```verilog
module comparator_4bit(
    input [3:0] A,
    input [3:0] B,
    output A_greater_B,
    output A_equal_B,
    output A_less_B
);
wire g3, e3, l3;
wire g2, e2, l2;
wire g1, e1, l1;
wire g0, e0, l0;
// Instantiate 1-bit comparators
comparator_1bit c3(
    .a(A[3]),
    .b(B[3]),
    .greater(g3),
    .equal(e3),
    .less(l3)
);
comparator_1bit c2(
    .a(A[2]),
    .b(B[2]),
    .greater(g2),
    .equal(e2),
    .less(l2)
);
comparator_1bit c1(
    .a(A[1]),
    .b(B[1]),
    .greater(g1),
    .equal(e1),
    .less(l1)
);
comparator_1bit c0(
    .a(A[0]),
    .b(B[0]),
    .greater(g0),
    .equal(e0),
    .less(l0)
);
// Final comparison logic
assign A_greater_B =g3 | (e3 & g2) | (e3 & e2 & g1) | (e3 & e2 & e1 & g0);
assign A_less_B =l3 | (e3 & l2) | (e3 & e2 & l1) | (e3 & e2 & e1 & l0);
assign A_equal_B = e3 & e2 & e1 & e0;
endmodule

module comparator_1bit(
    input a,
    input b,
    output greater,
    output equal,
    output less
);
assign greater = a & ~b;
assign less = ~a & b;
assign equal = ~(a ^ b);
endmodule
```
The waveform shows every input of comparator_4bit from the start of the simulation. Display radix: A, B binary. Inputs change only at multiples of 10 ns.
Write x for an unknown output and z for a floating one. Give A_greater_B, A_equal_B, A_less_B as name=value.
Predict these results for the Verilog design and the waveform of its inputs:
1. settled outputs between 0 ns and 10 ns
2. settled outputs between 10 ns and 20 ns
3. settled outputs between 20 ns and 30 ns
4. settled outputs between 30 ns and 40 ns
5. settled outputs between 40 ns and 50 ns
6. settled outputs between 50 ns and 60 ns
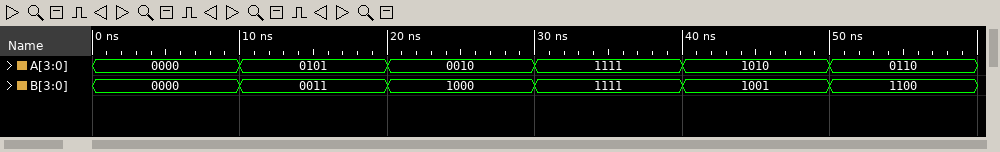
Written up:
A_greater_B=0, A_equal_B=1, A_less_B=0
A_greater_B=1, A_equal_B=0, A_less_B=0
A_greater_B=0, A_equal_B=0, A_less_B=1
A_greater_B=0, A_equal_B=1, A_less_B=0
A_greater_B=1, A_equal_B=0, A_less_B=0
A_greater_B=0, A_equal_B=0, A_less_B=1
